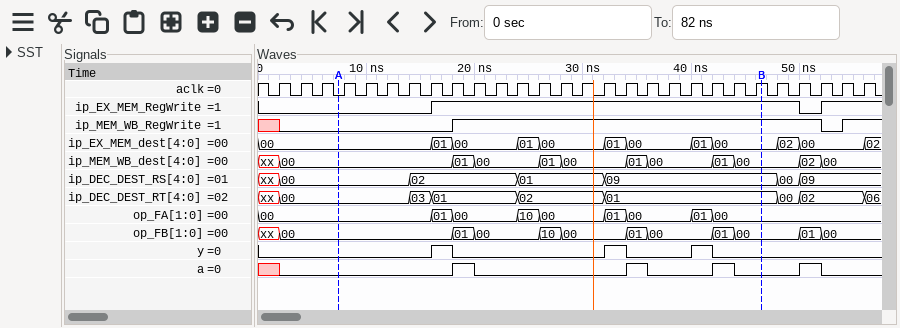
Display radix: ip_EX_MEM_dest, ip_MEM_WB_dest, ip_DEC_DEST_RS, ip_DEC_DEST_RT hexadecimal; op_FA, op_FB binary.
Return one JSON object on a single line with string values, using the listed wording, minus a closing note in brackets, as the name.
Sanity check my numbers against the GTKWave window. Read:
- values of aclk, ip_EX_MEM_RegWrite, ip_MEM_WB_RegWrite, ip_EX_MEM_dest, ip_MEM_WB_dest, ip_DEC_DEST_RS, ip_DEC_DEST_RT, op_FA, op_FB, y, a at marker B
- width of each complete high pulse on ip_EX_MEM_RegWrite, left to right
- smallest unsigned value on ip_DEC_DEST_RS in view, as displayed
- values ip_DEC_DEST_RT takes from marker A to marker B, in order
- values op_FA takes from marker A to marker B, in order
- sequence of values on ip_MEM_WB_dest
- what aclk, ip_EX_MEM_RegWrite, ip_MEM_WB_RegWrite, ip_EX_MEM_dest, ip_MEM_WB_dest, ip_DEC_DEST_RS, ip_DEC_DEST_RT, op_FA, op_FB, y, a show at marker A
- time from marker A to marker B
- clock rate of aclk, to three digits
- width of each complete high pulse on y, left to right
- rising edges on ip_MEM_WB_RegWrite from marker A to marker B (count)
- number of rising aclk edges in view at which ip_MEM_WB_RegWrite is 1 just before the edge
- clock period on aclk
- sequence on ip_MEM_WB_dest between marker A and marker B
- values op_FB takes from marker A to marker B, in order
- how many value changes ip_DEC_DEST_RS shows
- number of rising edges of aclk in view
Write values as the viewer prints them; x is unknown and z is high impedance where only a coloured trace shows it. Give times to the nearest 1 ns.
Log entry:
{"values of aclk, ip_EX_MEM_RegWrite, ip_MEM_WB_RegWrite, ip_EX_MEM_dest, ip_MEM_WB_dest, ip_DEC_DEST_RS, ip_DEC_DEST_RT, op_FA, op_FB, y, a at marker B": "aclk=1, ip_EX_MEM_RegWrite=1, ip_MEM_WB_RegWrite=1, ip_EX_MEM_dest=00, ip_MEM_WB_dest=00, ip_DEC_DEST_RS=09, ip_DEC_DEST_RT=01, op_FA=00, op_FB=00, y=0, a=0", "width of each complete high pulse on ip_EX_MEM_RegWrite, left to right": "34 ns", "smallest unsigned value on ip_DEC_DEST_RS in view, as displayed": "00", "values ip_DEC_DEST_RT takes from marker A to marker B, in order": "00, 03, 01, 02, 01", "values op_FA takes from marker A to marker B, in order": "00, 01, 00, 10, 00, 01, 00, 01, 00", "sequence of values on ip_MEM_WB_dest": "xx, 00, 01, 00, 01, 00, 01, 00, 01, 00, 02, 00", "what aclk, ip_EX_MEM_RegWrite, ip_MEM_WB_RegWrite, ip_EX_MEM_dest, ip_MEM_WB_dest, ip_DEC_DEST_RS, ip_DEC_DEST_RT, op_FA, op_FB, y, a show at marker A": "aclk=0, ip_EX_MEM_RegWrite=0, ip_MEM_WB_RegWrite=0, ip_EX_MEM_dest=00, ip_MEM_WB_dest=00, ip_DEC_DEST_RS=00, ip_DEC_DEST_RT=00, op_FA=00, op_FB=00, y=0, a=0", "time from marker A to marker B": "39 ns", "clock rate of aclk, to three digits": "500 MHz", "width of each complete high pulse on y, left to right": "2 ns, 2 ns, 2 ns", "rising edges on ip_MEM_WB_RegWrite from marker A to marker B": "1", "number of rising aclk edges in view at which ip_MEM_WB_RegWrite is 1 just before the edge": "18", "clock period on aclk": "2 ns", "sequence on ip_MEM_WB_dest between marker A and marker B": "00, 01, 00, 01, 00, 01, 00, 01, 00", "values op_FB takes from marker A to marker B, in order": "00, 01, 00, 10, 00, 01, 00, 01, 00", "how many value changes ip_DEC_DEST_RS shows": "6", "number of rising edges of aclk in view": "28"}
